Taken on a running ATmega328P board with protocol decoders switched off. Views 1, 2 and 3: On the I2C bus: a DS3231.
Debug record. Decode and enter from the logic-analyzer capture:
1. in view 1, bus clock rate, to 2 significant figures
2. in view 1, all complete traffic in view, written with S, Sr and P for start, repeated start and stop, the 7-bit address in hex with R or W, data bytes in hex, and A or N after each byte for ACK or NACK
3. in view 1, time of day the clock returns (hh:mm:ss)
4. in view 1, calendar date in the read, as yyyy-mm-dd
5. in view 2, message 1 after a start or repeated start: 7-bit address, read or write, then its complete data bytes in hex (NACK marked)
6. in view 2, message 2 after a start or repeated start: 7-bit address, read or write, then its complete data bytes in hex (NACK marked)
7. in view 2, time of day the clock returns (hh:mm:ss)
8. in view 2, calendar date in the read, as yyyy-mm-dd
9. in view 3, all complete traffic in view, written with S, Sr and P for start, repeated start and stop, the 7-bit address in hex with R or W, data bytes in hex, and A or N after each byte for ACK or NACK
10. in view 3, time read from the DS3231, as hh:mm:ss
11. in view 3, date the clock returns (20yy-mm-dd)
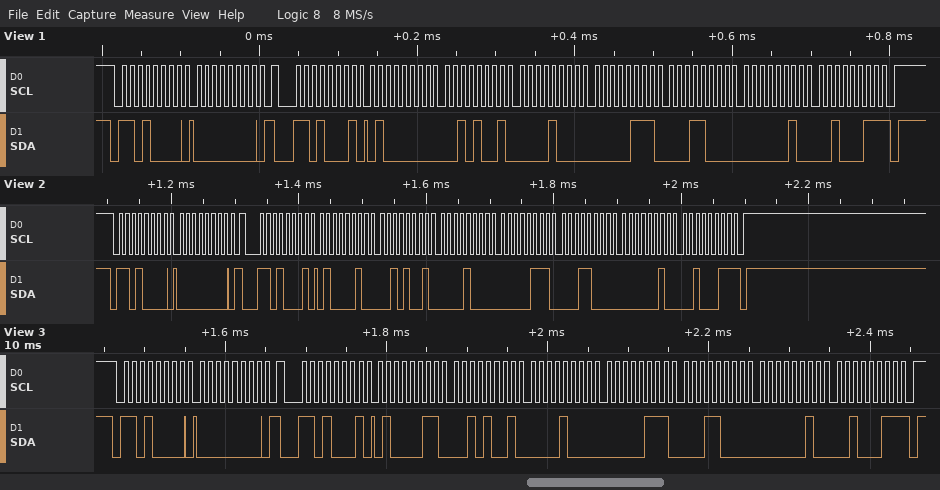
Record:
100 kHz
S 68W A 00 A Sr 68R A 40 A 29 A 08 A 07 A 18 A 02 A 23 N P
08:29:40
2023-02-18
0x68 write: 00
0x68 read: 42 29 08 07 18 02 23 NACK
08:29:42
2023-02-18
S 68W A 00 A Sr 68R A 43 A 29 A 08 A 07 A 18 A 02 A 23 N P
08:29:43
2023-02-18
